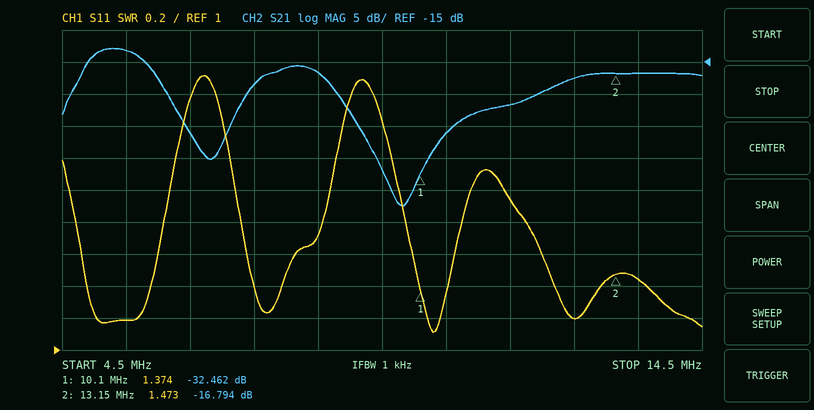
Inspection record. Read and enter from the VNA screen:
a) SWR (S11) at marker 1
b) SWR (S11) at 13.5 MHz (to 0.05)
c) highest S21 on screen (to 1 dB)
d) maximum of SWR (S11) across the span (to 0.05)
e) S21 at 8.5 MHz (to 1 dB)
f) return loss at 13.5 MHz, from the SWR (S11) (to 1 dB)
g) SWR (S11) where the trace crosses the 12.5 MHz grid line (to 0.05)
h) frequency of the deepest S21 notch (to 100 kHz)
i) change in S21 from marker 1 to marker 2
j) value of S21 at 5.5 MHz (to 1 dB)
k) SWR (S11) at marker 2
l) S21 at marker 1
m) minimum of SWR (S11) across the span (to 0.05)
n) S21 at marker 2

1.374
1.45
-13 dB
2.70
-17 dB
15 dB
1.20
9.8 MHz
15.668 dB
-13 dB
1.473
-32.462 dB
1.10
-16.794 dB
